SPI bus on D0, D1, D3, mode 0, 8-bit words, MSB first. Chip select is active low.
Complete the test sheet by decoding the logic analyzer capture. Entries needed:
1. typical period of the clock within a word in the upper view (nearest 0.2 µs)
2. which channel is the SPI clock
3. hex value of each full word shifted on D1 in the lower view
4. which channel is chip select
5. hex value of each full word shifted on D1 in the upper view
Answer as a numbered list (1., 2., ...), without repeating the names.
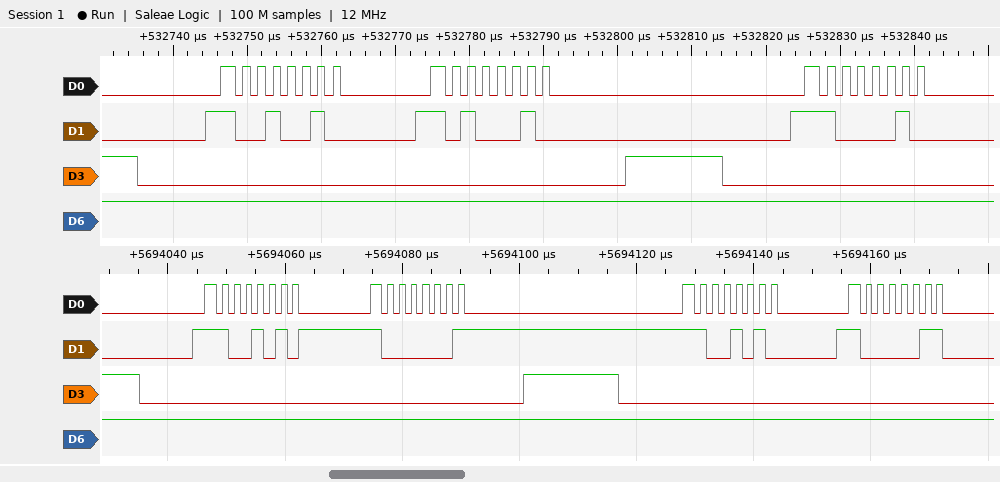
1. 2 µs
2. D0
3. CA, 81, CA, 83
4. D3
5. 92, A2, C2
